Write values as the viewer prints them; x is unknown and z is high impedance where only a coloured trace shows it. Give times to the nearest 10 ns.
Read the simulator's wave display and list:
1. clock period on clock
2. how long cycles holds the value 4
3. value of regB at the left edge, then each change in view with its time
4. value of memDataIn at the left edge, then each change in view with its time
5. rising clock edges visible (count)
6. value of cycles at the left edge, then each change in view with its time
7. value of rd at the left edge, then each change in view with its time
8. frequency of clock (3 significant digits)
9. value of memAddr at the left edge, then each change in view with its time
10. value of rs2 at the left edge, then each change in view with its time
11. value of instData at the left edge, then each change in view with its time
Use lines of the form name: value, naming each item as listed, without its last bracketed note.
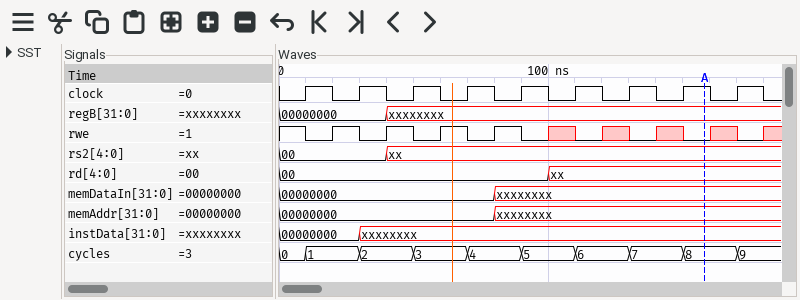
clock period on clock: 20 ns
how long cycles holds the value 4: 20 ns
value of regB at the left edge, then each change in view with its time: 00000000, xxxxxxxx at 40 ns
value of memDataIn at the left edge, then each change in view with its time: 00000000, xxxxxxxx at 80 ns
rising clock edges visible: 9
value of cycles at the left edge, then each change in view with its time: 0, 1 at 10 ns, 2 at 30 ns, 3 at 50 ns, 4 at 70 ns, 5 at 90 ns, 6 at 110 ns, 7 at 130 ns, 8 at 150 ns, 9 at 170 ns
value of rd at the left edge, then each change in view with its time: 00, xx at 100 ns
frequency of clock: 50.0 MHz
value of memAddr at the left edge, then each change in view with its time: 00000000, xxxxxxxx at 80 ns
value of rs2 at the left edge, then each change in view with its time: 00, xx at 40 ns
value of instData at the left edge, then each change in view with its time: 00000000, xxxxxxxx at 30 ns
